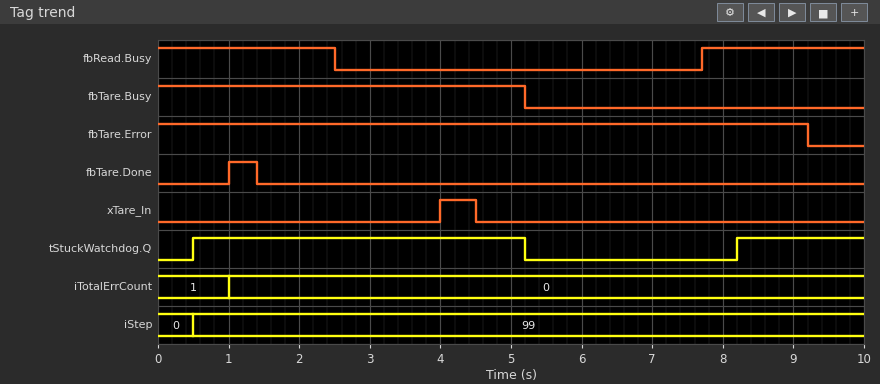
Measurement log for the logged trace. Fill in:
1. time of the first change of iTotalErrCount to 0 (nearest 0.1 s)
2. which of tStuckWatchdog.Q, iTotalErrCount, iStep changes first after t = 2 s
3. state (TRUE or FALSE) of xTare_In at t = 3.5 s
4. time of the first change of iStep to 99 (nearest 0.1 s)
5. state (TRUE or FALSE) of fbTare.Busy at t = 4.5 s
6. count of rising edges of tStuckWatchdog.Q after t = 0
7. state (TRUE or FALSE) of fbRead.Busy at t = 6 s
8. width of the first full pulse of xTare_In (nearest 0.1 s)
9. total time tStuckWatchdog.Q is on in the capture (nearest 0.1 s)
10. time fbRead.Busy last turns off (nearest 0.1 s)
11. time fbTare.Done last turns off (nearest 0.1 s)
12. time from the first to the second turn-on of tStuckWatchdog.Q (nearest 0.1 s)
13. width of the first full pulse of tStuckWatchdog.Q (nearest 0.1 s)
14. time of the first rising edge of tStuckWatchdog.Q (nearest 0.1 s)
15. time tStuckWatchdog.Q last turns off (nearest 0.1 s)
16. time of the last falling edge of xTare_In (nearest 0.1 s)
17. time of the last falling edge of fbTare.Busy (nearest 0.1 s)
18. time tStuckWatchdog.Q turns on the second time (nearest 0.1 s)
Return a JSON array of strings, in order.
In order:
["1.0 s", "tStuckWatchdog.Q", "FALSE", "0.5 s", "TRUE", "2", "FALSE", "0.5 s", "6.5 s", "2.5 s", "1.4 s", "7.7 s", "4.7 s", "0.5 s", "5.2 s", "4.5 s", "5.2 s", "8.2 s"]
